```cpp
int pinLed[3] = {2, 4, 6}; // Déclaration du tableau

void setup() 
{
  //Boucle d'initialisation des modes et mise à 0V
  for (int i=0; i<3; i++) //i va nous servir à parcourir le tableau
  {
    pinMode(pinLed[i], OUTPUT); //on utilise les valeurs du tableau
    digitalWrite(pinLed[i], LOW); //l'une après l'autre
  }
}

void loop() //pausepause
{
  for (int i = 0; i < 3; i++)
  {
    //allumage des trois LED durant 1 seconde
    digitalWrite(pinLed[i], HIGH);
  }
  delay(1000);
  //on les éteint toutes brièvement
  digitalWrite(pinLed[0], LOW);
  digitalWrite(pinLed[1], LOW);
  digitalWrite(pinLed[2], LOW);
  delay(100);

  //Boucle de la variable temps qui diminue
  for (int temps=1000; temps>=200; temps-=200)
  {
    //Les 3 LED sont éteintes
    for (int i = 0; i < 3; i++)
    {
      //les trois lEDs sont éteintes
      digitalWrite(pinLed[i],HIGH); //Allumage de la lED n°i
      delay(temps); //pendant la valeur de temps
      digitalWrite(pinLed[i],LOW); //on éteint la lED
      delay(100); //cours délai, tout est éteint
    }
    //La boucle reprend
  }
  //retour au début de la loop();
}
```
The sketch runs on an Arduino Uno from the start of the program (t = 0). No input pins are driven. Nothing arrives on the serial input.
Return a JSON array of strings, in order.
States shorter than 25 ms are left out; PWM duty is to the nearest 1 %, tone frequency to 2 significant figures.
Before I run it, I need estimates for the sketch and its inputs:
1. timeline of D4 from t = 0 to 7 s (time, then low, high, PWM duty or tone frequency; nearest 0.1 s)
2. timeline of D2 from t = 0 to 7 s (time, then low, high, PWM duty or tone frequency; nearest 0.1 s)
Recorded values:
["0 s high; 1 s low; 2.2 s high; 3.2 s low; 5.3 s high; 6.1 s low", "0 s high; 1 s low; 1.1 s high; 2.1 s low; 4.4 s high; 5.2 s low"]
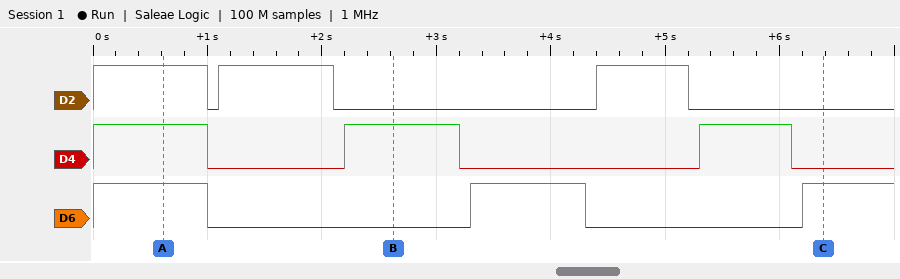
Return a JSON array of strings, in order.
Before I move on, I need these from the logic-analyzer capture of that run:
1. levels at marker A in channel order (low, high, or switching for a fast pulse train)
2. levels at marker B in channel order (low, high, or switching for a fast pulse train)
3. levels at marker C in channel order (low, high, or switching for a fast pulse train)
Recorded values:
["D2 high, D4 high, D6 high", "D2 low, D4 high, D6 low", "D2 low, D4 low, D6 high"]
